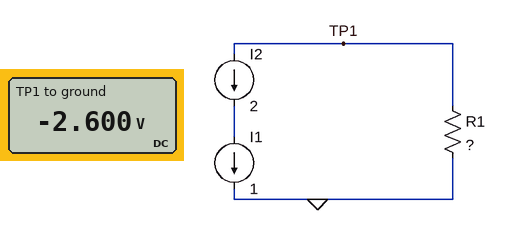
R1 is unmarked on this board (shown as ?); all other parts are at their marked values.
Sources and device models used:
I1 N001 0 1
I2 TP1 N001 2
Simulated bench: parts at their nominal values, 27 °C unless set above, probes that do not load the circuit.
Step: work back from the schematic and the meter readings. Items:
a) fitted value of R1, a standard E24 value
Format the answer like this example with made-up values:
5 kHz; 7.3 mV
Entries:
1.3 Ω
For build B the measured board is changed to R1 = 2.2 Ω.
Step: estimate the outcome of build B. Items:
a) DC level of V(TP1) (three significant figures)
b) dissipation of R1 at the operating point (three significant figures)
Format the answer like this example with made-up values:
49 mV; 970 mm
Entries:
-4.40 V; 8.80 W
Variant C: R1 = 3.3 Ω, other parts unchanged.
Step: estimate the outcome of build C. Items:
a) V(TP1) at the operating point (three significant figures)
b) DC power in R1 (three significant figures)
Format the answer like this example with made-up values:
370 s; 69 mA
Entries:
-6.60 V; 13.2 W
